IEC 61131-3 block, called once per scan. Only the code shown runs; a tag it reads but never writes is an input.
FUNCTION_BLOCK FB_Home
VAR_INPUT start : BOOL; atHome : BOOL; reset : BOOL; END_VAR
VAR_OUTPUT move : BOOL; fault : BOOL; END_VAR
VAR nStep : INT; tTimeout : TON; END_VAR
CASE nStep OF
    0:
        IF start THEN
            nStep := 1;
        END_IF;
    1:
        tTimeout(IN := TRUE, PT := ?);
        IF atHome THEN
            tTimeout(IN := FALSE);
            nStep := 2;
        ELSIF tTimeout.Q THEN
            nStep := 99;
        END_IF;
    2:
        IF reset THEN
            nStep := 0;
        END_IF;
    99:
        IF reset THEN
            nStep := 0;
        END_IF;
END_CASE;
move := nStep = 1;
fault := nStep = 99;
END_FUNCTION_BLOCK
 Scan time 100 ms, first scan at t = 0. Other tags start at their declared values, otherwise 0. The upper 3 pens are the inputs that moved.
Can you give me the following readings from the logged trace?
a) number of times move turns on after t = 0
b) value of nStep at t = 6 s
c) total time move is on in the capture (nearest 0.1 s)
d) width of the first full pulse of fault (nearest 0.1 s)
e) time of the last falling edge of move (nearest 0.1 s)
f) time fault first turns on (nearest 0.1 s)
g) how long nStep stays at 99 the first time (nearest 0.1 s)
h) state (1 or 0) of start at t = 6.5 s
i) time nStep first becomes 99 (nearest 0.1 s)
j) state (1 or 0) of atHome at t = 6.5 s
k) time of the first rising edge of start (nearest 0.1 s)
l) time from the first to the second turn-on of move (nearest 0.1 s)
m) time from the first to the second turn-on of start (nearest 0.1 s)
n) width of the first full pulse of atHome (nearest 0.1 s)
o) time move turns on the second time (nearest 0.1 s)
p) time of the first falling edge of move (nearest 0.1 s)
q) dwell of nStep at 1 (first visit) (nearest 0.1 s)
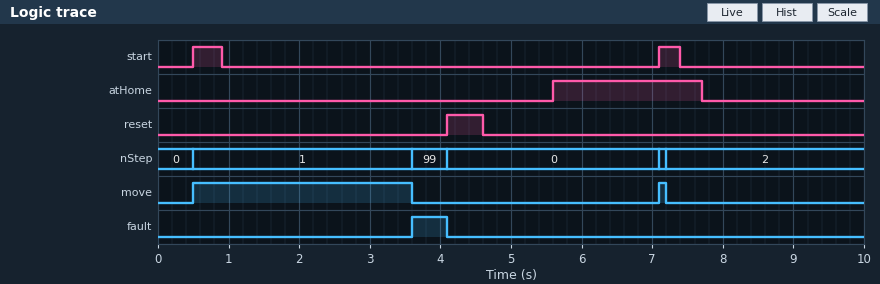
2
0
3.2 s
0.5 s
7.2 s
3.6 s
0.5 s
0
3.6 s
1
0.5 s
6.6 s
6.6 s
2.1 s
7.1 s
3.6 s
3.1 s
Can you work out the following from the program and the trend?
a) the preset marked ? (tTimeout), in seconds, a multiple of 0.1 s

3.0 s
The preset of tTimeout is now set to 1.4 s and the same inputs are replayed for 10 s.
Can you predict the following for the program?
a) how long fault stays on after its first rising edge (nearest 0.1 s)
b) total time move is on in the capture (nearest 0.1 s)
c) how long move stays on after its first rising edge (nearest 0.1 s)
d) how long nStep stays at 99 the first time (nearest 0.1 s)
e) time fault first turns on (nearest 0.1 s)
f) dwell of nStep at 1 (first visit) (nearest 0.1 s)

2.1 s
1.6 s
1.5 s
2.1 s
2.0 s
1.5 s
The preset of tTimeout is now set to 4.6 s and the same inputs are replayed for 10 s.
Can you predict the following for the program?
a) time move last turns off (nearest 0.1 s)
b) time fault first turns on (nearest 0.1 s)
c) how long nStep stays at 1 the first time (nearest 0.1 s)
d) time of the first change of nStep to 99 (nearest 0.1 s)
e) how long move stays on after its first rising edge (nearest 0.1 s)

5.2 s
5.2 s
4.7 s
5.2 s
4.7 s
